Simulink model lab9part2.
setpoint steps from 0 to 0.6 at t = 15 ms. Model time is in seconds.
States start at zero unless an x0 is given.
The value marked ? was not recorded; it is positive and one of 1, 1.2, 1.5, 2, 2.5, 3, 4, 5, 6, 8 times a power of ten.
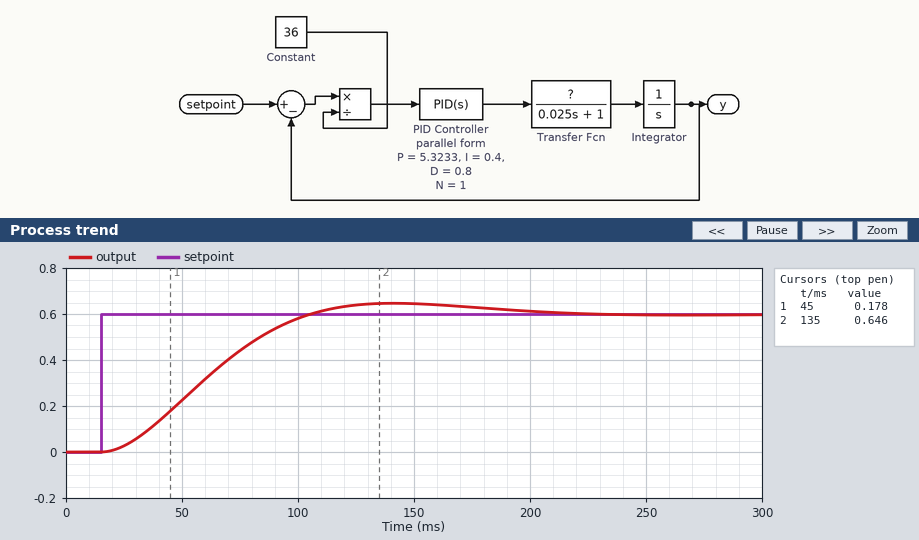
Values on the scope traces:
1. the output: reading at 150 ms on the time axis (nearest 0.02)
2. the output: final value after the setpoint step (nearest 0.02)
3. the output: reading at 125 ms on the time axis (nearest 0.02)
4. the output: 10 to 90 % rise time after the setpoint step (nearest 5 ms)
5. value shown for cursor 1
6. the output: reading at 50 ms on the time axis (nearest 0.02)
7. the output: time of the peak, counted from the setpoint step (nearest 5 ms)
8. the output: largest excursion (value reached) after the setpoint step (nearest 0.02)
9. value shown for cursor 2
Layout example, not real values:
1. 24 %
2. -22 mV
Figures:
1. 0.64
2. 0.60
3. 0.64
4. 60 ms
5. 0.178
6. 0.22
7. 125 ms
8. 0.64
9. 0.646
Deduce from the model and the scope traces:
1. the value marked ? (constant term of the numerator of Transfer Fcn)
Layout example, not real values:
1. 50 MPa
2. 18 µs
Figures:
1. 150
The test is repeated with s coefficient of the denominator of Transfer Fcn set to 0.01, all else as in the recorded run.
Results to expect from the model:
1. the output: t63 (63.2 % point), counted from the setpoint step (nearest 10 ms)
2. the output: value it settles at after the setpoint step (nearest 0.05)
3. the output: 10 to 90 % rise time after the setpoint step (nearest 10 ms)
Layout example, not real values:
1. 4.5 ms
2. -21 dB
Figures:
1. 40 ms
2. 0.60
3. 70 ms
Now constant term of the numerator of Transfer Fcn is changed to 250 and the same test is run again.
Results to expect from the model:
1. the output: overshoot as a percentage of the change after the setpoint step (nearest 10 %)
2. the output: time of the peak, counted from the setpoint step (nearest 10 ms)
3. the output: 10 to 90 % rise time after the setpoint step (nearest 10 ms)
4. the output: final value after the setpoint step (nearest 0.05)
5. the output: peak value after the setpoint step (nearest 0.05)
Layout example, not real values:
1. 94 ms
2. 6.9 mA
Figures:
1. 20 %
2. 90 ms
3. 40 ms
4. 0.60
5. 0.70
